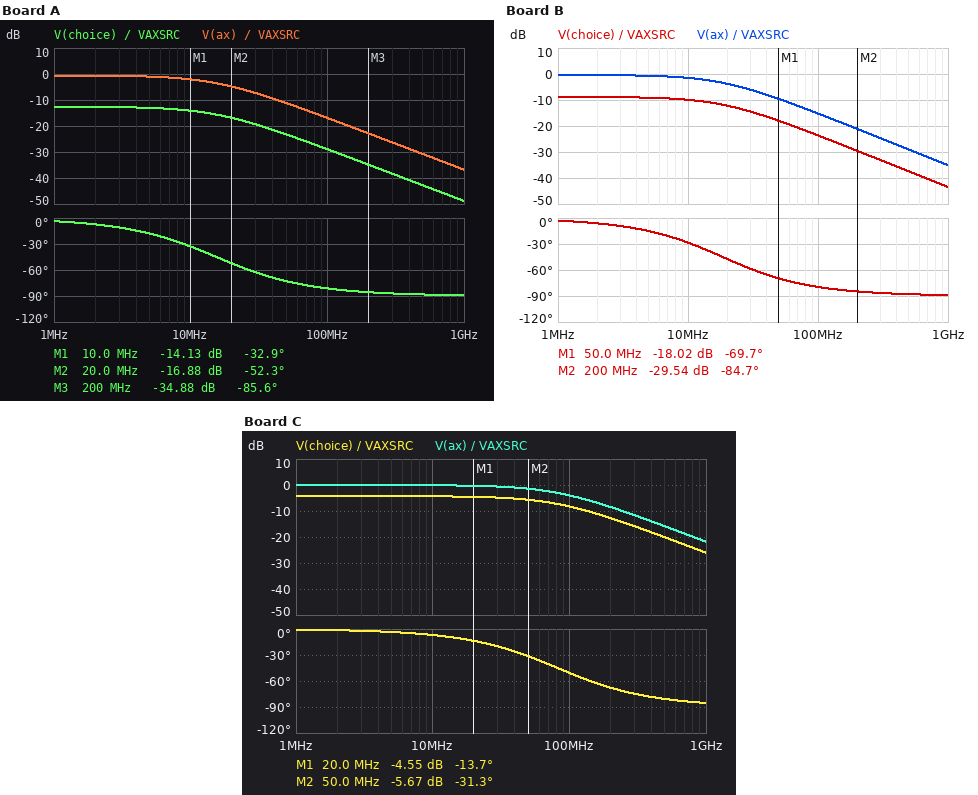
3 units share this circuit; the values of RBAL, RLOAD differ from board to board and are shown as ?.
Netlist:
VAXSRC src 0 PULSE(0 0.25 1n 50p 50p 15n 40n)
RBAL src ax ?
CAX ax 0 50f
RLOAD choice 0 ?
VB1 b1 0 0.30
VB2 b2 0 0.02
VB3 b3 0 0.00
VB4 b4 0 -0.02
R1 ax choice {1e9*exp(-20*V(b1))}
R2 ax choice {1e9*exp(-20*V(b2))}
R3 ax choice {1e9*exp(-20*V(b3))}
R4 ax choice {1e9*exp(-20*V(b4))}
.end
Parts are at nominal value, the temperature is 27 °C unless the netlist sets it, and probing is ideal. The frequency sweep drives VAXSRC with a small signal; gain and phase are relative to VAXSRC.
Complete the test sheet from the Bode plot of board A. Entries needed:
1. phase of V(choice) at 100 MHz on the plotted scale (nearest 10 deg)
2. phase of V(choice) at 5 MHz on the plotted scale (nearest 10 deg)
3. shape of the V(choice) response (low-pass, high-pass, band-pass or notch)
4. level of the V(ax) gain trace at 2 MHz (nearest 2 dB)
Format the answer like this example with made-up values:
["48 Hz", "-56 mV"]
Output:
["-80 deg", "-20 deg", "low-pass", "0 dB"]
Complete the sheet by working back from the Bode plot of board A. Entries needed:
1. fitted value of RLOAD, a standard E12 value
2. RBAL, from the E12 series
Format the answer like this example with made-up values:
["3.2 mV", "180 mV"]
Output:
["820 kΩ", "220 kΩ"]
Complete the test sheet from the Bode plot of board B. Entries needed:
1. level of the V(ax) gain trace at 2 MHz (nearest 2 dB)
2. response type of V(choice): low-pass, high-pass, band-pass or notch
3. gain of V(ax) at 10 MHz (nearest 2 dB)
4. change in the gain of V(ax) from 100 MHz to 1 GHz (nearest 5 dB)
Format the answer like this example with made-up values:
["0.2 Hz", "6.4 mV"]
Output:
["0 dB", "low-pass", "-2 dB", "-20 dB"]
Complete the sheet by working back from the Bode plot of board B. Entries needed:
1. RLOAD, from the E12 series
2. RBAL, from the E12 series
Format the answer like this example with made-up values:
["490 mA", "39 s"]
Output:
["1.5 MΩ", "180 kΩ"]
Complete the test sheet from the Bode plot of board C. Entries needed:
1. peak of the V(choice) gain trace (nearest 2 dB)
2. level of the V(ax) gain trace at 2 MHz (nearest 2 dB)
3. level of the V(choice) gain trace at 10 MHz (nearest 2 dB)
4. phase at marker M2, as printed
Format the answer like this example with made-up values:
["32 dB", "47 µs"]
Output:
["-4 dB", "0 dB", "-4 dB", "-31.3 deg"]
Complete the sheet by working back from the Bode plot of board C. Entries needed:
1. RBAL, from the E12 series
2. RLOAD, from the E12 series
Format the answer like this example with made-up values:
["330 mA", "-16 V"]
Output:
["39 kΩ", "3.9 MΩ"]
